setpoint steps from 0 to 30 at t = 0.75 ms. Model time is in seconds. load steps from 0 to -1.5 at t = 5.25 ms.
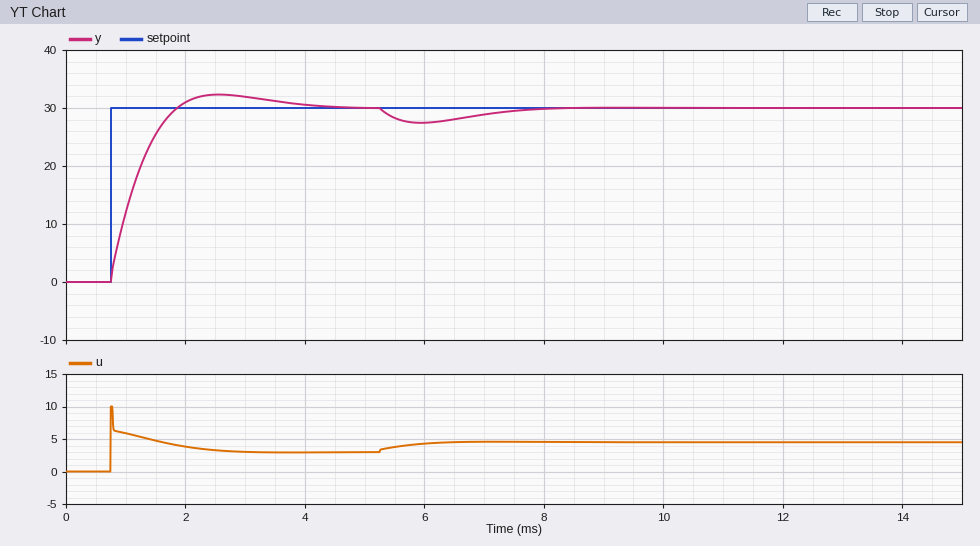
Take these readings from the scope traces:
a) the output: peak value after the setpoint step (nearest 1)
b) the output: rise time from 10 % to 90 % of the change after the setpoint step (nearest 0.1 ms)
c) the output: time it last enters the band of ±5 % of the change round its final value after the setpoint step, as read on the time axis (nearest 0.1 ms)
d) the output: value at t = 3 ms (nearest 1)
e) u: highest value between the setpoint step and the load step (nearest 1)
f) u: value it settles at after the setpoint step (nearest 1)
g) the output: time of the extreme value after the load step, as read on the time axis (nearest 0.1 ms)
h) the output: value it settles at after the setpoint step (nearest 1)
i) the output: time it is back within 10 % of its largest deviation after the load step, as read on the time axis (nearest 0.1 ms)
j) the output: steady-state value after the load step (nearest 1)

32
0.8 ms
3.3 ms
32
10
3
5.9 ms
30
7.8 ms
30
